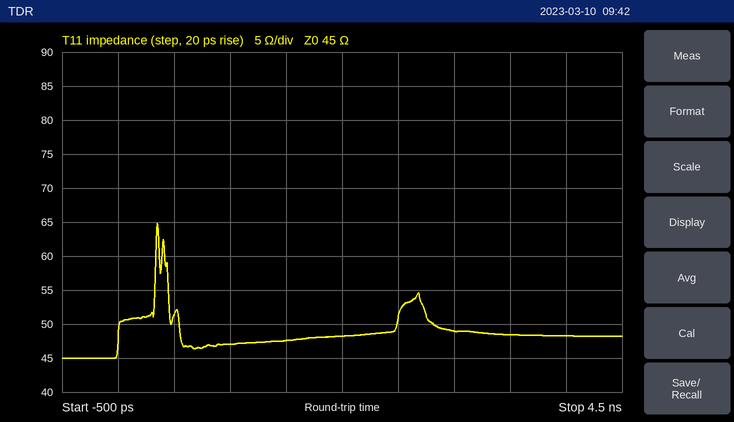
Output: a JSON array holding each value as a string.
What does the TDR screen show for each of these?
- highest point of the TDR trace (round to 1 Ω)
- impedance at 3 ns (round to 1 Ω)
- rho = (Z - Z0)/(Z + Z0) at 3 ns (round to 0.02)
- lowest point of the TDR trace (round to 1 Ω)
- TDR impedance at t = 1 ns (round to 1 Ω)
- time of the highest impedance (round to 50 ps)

["65 Ω", "49 Ω", "+0.04", "45 Ω", "47 Ω", "350 ps"]
